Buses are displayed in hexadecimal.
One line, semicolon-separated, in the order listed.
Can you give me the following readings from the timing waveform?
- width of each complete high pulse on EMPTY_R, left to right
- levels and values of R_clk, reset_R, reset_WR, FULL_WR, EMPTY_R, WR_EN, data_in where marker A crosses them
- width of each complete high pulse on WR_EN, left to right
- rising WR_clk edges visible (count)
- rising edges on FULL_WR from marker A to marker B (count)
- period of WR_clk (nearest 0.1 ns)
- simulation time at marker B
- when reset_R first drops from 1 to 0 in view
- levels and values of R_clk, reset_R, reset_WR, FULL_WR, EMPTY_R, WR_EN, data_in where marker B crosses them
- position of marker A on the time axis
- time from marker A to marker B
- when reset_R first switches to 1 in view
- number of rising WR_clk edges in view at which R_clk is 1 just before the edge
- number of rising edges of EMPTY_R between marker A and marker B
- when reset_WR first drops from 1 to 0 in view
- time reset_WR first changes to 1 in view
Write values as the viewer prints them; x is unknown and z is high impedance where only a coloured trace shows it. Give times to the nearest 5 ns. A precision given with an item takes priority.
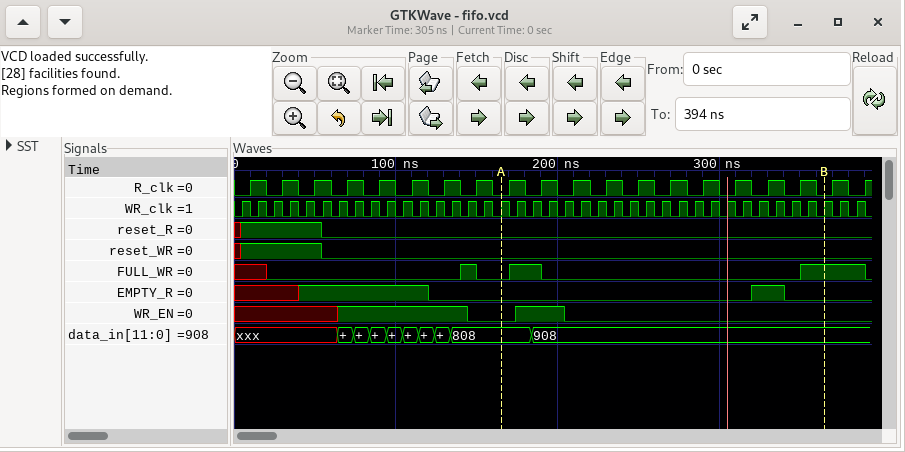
20 ns; R_clk=0, reset_R=0, reset_WR=0, FULL_WR=0, EMPTY_R=0, WR_EN=0, data_in=808; 30 ns; 39; 2; 10 ns; 365 ns; 55 ns; R_clk=0, reset_R=0, reset_WR=0, FULL_WR=1, EMPTY_R=0, WR_EN=0, data_in=908; 165 ns; 200 ns; 5 ns; 19; 1; 55 ns; 5 ns
